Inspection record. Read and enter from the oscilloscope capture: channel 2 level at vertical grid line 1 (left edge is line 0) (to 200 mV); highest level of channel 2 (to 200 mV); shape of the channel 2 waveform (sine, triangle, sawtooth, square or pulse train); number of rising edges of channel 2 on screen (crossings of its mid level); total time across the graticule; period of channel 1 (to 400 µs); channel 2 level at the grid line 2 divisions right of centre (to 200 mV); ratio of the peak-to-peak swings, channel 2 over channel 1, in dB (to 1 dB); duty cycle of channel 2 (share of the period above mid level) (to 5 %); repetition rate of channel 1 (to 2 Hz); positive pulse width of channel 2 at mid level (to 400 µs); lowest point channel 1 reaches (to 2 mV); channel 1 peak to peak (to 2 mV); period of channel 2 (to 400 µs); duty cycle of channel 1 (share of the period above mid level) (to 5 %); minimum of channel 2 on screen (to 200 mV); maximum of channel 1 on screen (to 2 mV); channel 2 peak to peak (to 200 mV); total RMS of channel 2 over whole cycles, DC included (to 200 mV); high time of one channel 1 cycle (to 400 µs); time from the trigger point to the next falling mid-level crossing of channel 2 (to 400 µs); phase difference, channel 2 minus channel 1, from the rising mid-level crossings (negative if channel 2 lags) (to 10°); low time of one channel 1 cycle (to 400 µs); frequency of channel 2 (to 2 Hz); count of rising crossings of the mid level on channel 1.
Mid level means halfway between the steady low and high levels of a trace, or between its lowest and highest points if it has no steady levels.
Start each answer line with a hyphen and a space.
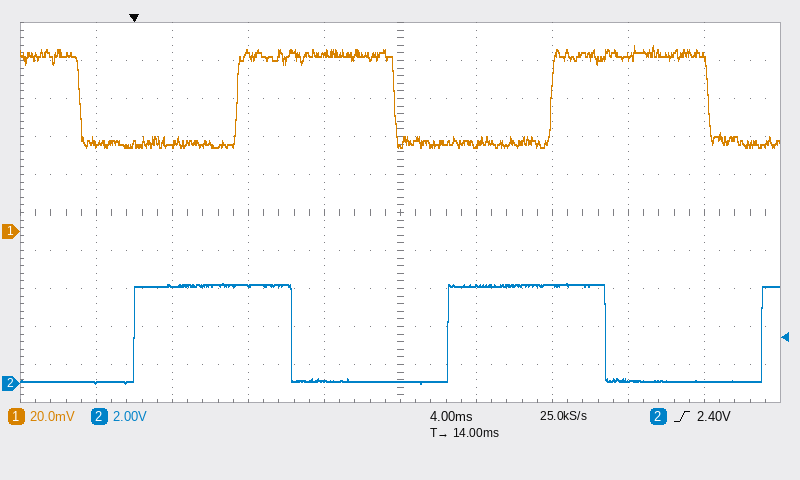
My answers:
- 0.0 V
- 5.2 V
- square
- 3
- 40 ms
- 16.4 ms
- 5.2 V
- 40 dB
- 50 %
- 60 Hz
- 8.4 ms
- 44 mV
- 54 mV
- 16.4 ms
- 50 %
- 0.0 V
- 98 mV
- 5.2 V
- 3.6 V
- 8.4 ms
- 8.4 ms
- +120°
- 8.4 ms
- 60 Hz
- 2
